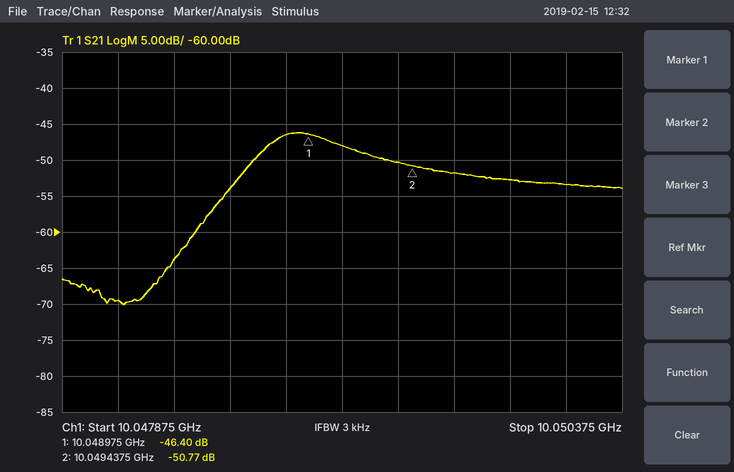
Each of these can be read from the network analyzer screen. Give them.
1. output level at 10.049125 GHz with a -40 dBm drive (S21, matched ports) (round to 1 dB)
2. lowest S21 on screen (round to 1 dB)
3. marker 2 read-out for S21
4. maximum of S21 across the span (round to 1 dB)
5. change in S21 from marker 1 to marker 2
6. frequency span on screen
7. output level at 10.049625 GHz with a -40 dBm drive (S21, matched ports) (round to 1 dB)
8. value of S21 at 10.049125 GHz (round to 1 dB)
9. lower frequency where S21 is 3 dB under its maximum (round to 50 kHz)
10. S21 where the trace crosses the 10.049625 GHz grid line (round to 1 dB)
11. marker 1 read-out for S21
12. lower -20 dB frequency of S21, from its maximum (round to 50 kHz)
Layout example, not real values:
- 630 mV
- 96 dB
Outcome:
- -88 dBm
- -70 dB
- -50.77 dB
- -46 dB
- -4.37 dB
- 2.5 MHz
- -92 dBm
- -48 dB
- 10.04875 GHz
- -52 dB
- -46.40 dB
- 10.04830 GHz
